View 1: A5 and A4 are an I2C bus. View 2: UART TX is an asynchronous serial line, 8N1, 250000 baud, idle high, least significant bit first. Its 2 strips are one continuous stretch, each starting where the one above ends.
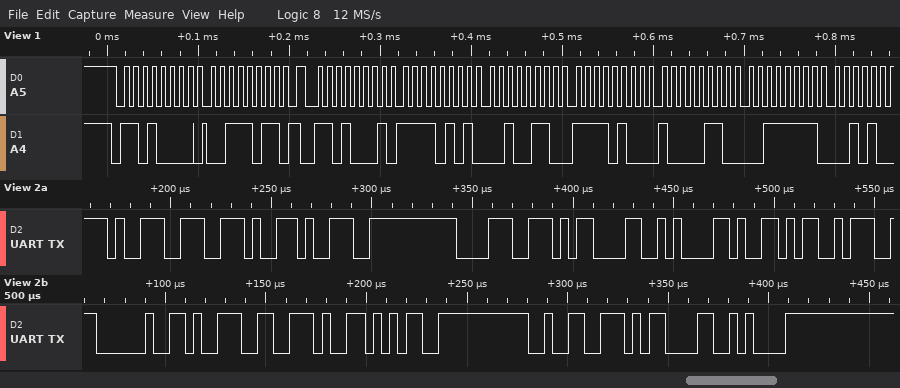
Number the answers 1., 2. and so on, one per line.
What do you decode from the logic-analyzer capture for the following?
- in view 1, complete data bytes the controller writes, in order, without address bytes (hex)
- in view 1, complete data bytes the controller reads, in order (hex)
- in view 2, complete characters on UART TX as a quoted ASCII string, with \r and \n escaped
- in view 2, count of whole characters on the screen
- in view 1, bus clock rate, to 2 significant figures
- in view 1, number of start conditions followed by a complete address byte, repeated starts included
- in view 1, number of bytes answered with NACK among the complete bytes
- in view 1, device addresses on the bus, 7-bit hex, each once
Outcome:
1. 3B
2. F5 26 F4 86 3F
3. "9.98\r\nY: 9.52\r\n"
4. 15
5. 100 kHz
6. 2
7. 0
8. 0x68
